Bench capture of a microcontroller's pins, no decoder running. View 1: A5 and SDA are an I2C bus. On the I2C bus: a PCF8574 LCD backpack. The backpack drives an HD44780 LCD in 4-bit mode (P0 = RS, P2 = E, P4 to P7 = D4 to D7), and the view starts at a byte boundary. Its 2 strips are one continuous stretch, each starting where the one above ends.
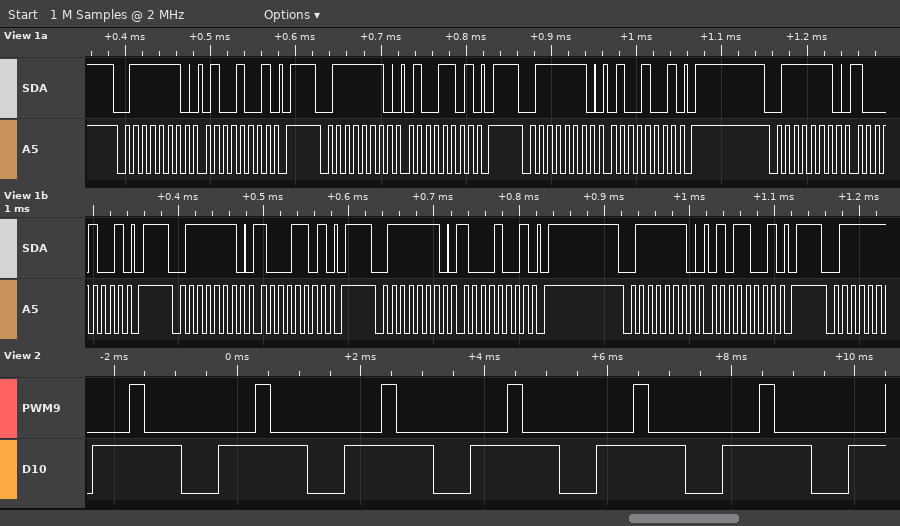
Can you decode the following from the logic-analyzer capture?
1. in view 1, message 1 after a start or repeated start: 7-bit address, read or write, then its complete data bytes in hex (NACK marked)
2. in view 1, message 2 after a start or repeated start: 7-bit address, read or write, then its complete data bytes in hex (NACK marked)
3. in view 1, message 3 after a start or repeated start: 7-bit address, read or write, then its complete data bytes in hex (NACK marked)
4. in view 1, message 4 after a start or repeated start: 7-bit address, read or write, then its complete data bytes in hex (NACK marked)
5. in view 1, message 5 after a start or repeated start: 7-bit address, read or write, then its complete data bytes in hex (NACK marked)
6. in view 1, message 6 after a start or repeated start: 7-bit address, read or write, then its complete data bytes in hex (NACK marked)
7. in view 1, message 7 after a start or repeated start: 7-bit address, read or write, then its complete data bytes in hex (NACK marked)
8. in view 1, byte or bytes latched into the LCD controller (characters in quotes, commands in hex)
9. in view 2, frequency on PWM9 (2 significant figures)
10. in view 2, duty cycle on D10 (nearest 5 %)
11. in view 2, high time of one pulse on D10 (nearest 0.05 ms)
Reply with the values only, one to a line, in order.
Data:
0x3F write: 49
0x3F write: 4D
0x3F write: 49
0x3F write: 89
0x3F write: 8D
0x3F write: 89
0x3F write: 59
'H'
490 Hz
70 %
1.45 ms
